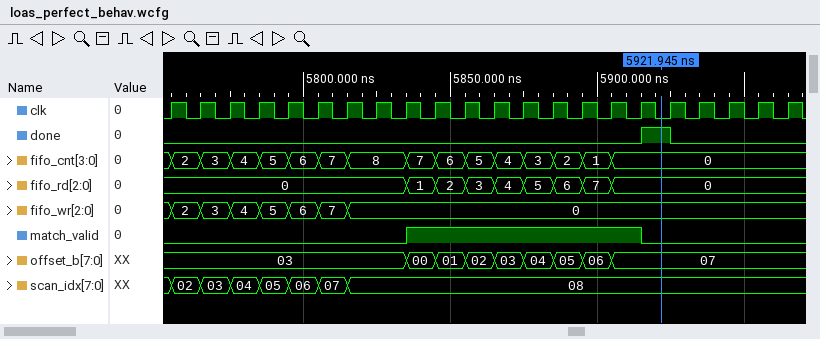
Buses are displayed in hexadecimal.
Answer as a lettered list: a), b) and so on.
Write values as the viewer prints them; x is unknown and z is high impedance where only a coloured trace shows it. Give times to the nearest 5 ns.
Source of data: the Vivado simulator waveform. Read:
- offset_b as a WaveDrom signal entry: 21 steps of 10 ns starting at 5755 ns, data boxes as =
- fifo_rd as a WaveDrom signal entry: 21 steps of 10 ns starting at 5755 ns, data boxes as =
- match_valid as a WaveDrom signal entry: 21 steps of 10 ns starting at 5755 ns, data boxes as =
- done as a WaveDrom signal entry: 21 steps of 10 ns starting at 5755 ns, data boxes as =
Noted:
a) {name: 'offset_b', wave: '=.......========.....', data: '03 00 01 02 03 04 05 06 07'}
b) {name: 'fifo_rd', wave: '=.......========.....', data: '0 1 2 3 4 5 6 7 0'}
c) {name: 'match_valid', wave: '0.......1.......0....'}
d) {name: 'done', wave: '0...............10...'}
